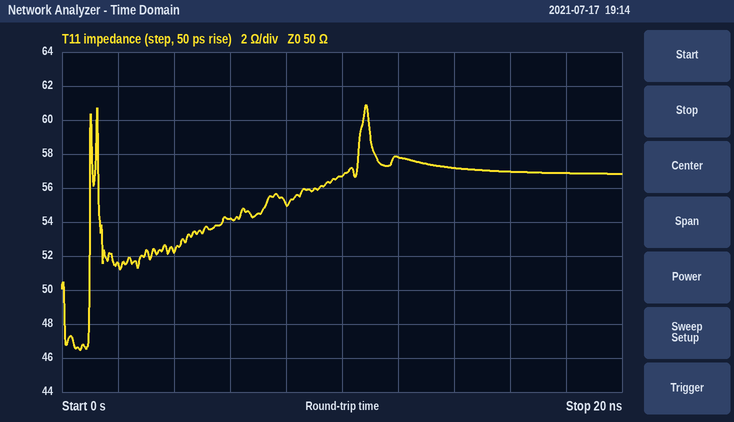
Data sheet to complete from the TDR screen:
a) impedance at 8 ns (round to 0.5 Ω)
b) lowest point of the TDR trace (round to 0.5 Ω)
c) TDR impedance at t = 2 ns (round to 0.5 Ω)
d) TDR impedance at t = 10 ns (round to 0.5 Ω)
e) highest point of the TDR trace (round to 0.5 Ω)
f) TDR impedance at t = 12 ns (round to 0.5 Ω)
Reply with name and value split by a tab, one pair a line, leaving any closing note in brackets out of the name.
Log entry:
impedance at 8 ns	55.0 Ω
lowest point of the TDR trace	46.5 Ω
TDR impedance at t = 2 ns	51.5 Ω
TDR impedance at t = 10 ns	56.5 Ω
highest point of the TDR trace	61.0 Ω
TDR impedance at t = 12 ns	58.0 Ω
